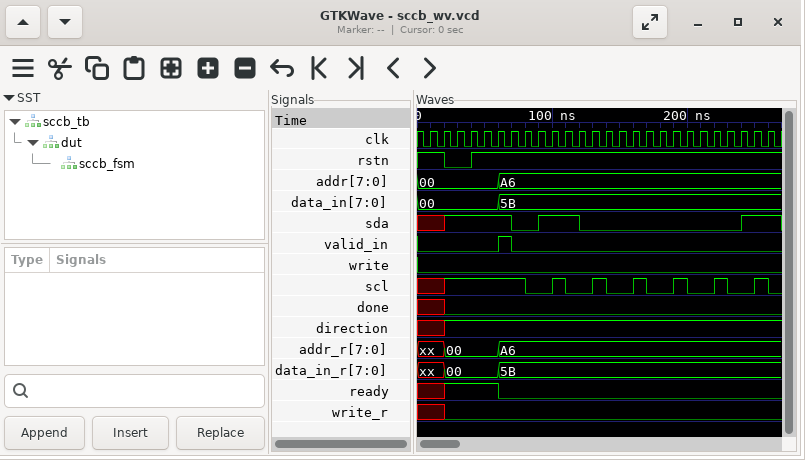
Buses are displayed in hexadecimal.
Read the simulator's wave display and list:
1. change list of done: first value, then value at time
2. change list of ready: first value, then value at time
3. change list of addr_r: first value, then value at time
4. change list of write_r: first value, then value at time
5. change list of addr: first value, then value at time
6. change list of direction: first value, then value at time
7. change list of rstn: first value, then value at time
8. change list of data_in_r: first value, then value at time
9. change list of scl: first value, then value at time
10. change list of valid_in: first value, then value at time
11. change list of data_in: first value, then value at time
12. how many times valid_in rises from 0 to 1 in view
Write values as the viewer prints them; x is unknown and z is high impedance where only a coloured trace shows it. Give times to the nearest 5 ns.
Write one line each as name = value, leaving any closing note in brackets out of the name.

change list of done: first value, then value at time = x, 0 at 20 ns
change list of ready: first value, then value at time = x, 1 at 20 ns, 0 at 60 ns
change list of addr_r: first value, then value at time = xx, 00 at 20 ns, A6 at 60 ns
change list of write_r: first value, then value at time = x, 0 at 20 ns
change list of addr: first value, then value at time = 00, A6 at 60 ns
change list of direction: first value, then value at time = x, 1 at 20 ns
change list of rstn: first value, then value at time = 1, 0 at 20 ns, 1 at 40 ns
change list of data_in_r: first value, then value at time = xx, 00 at 20 ns, 5B at 60 ns
change list of scl: first value, then value at time = x, 1 at 20 ns, 0 at 80 ns, 1 at 100 ns, 0 at 110 ns, 1 at 130 ns, 0 at 140 ns, 1 at 160 ns, 0 at 170 ns, 1 at 190 ns, 0 at 200 ns, 1 at 220 ns, 0 at 230 ns, 1 at 250 ns, 0 at 260 ns
change list of valid_in: first value, then value at time = 0, 1 at 60 ns, 0 at 70 ns
change list of data_in: first value, then value at time = 00, 5B at 60 ns
how many times valid_in rises from 0 to 1 in view = 1
